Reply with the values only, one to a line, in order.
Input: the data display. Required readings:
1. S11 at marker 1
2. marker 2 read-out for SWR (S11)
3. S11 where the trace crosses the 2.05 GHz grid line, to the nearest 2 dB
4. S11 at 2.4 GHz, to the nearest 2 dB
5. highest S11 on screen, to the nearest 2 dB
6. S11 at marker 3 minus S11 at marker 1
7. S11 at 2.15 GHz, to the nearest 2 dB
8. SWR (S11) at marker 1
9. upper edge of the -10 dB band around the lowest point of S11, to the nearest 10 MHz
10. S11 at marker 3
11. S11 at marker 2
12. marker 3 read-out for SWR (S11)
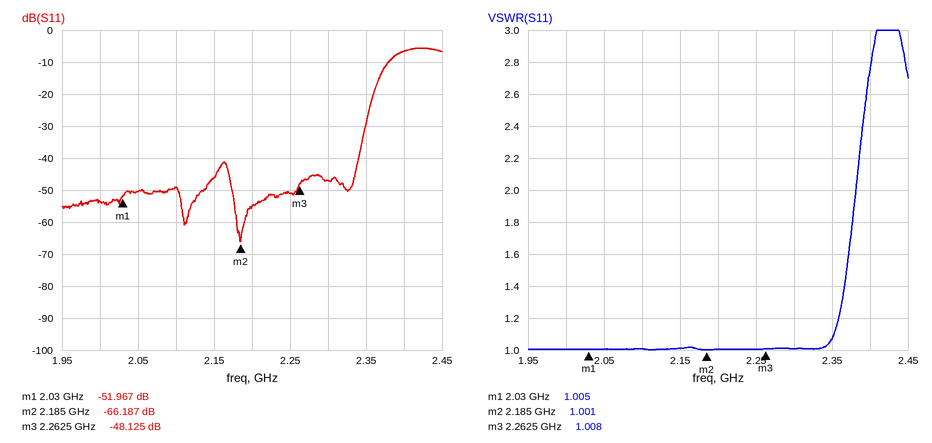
-51.967 dB
1.001
-50 dB
-6 dB
-6 dB
3.842 dB
-46 dB
1.005
2.38 GHz
-48.125 dB
-66.187 dB
1.008
